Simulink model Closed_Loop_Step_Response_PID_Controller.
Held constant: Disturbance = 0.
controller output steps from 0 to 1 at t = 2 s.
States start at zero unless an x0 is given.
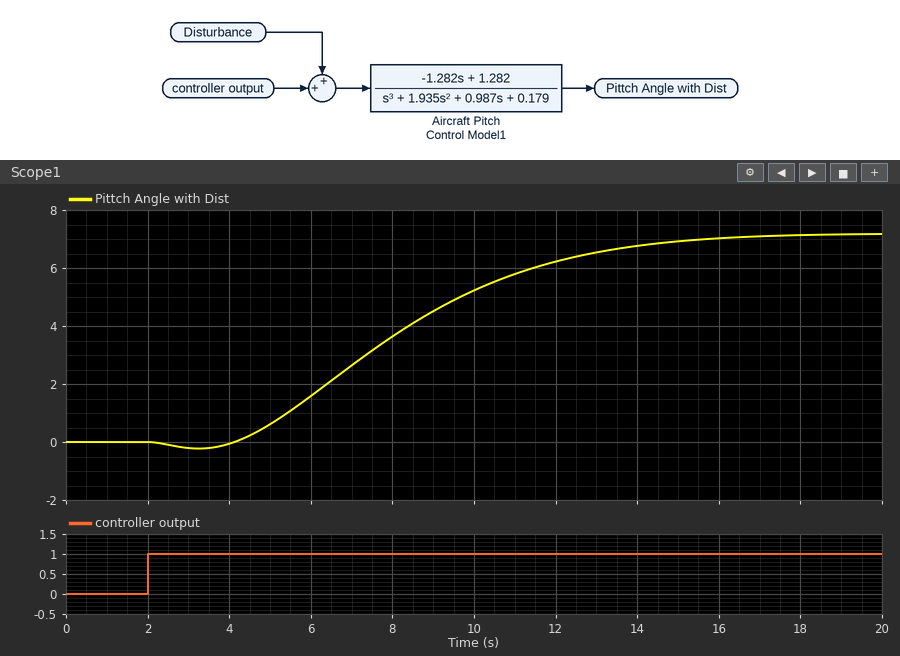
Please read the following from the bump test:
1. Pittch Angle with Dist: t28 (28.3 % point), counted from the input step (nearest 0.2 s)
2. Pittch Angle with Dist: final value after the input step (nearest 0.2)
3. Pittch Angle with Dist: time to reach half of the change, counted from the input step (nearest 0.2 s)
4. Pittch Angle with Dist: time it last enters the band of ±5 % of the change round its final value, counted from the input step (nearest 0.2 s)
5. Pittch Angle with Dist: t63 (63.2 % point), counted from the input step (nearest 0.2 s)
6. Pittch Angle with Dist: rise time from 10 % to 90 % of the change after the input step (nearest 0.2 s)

4.4 s
7.2
6.0 s
12.2 s
7.0 s
7.6 s
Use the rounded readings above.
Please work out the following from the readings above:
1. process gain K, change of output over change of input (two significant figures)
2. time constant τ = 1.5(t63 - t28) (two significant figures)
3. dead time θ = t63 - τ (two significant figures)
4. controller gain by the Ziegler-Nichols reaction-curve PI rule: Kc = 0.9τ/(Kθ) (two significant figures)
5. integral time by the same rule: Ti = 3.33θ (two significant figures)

7.2
3.9 s
3.1 s
0.16
10 s
